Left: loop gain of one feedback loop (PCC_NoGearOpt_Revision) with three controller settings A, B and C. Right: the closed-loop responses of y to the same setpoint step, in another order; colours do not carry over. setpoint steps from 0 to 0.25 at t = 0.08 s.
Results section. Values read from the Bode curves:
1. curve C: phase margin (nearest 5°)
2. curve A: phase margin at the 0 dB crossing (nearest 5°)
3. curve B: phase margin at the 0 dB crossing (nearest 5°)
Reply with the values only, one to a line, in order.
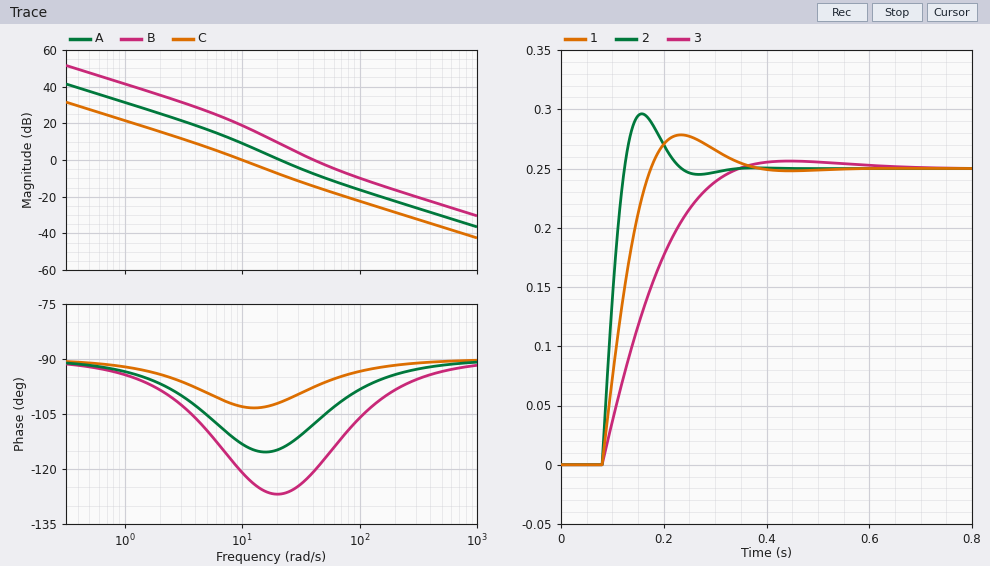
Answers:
75°
65°
60°
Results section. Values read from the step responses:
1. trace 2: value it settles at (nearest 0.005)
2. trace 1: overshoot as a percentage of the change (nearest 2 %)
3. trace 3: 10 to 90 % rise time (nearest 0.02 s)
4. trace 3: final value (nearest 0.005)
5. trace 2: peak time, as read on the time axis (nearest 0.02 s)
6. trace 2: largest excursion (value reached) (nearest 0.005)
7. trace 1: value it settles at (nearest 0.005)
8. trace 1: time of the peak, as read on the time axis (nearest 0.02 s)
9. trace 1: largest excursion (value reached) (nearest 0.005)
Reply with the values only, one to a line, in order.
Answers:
0.250
12 %
0.18 s
0.250
0.16 s
0.295
0.250
0.24 s
0.280
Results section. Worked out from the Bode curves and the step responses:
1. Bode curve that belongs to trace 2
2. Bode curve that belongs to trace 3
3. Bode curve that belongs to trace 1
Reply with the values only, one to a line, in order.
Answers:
B
C
A
